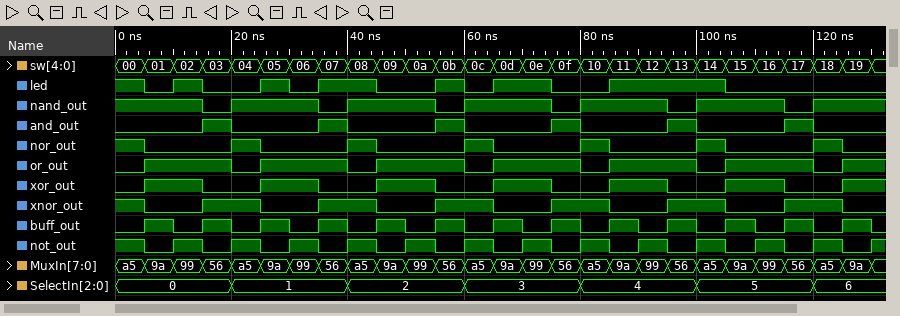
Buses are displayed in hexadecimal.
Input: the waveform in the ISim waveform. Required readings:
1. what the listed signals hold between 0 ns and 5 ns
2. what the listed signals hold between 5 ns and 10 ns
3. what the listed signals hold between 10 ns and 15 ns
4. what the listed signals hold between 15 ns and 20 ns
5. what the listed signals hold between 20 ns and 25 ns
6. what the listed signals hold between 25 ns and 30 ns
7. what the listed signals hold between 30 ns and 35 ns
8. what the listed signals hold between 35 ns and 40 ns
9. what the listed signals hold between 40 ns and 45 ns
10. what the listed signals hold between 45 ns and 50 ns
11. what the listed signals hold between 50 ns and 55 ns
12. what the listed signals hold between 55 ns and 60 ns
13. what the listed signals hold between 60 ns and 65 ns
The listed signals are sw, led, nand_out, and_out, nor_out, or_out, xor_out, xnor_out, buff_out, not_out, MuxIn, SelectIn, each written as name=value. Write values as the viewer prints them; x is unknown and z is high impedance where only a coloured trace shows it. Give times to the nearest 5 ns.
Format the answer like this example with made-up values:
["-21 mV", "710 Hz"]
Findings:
["sw=00, led=1, nand_out=1, and_out=0, nor_out=1, or_out=0, xor_out=0, xnor_out=1, buff_out=0, not_out=1, MuxIn=a5, SelectIn=0", "sw=01, led=0, nand_out=1, and_out=0, nor_out=0, or_out=1, xor_out=1, xnor_out=0, buff_out=1, not_out=0, MuxIn=9a, SelectIn=0", "sw=02, led=1, nand_out=1, and_out=0, nor_out=0, or_out=1, xor_out=1, xnor_out=0, buff_out=0, not_out=1, MuxIn=99, SelectIn=0", "sw=03, led=0, nand_out=0, and_out=1, nor_out=0, or_out=1, xor_out=0, xnor_out=1, buff_out=1, not_out=0, MuxIn=56, SelectIn=0", "sw=04, led=0, nand_out=1, and_out=0, nor_out=1, or_out=0, xor_out=0, xnor_out=1, buff_out=0, not_out=1, MuxIn=a5, SelectIn=1", "sw=05, led=1, nand_out=1, and_out=0, nor_out=0, or_out=1, xor_out=1, xnor_out=0, buff_out=1, not_out=0, MuxIn=9a, SelectIn=1", "sw=06, led=0, nand_out=1, and_out=0, nor_out=0, or_out=1, xor_out=1, xnor_out=0, buff_out=0, not_out=1, MuxIn=99, SelectIn=1", "sw=07, led=1, nand_out=0, and_out=1, nor_out=0, or_out=1, xor_out=0, xnor_out=1, buff_out=1, not_out=0, MuxIn=56, SelectIn=1", "sw=08, led=1, nand_out=1, and_out=0, nor_out=1, or_out=0, xor_out=0, xnor_out=1, buff_out=0, not_out=1, MuxIn=a5, SelectIn=2", "sw=09, led=0, nand_out=1, and_out=0, nor_out=0, or_out=1, xor_out=1, xnor_out=0, buff_out=1, not_out=0, MuxIn=9a, SelectIn=2", "sw=0a, led=0, nand_out=1, and_out=0, nor_out=0, or_out=1, xor_out=1, xnor_out=0, buff_out=0, not_out=1, MuxIn=99, SelectIn=2", "sw=0b, led=1, nand_out=0, and_out=1, nor_out=0, or_out=1, xor_out=0, xnor_out=1, buff_out=1, not_out=0, MuxIn=56, SelectIn=2", "sw=0c, led=0, nand_out=1, and_out=0, nor_out=1, or_out=0, xor_out=0, xnor_out=1, buff_out=0, not_out=1, MuxIn=a5, SelectIn=3"]
